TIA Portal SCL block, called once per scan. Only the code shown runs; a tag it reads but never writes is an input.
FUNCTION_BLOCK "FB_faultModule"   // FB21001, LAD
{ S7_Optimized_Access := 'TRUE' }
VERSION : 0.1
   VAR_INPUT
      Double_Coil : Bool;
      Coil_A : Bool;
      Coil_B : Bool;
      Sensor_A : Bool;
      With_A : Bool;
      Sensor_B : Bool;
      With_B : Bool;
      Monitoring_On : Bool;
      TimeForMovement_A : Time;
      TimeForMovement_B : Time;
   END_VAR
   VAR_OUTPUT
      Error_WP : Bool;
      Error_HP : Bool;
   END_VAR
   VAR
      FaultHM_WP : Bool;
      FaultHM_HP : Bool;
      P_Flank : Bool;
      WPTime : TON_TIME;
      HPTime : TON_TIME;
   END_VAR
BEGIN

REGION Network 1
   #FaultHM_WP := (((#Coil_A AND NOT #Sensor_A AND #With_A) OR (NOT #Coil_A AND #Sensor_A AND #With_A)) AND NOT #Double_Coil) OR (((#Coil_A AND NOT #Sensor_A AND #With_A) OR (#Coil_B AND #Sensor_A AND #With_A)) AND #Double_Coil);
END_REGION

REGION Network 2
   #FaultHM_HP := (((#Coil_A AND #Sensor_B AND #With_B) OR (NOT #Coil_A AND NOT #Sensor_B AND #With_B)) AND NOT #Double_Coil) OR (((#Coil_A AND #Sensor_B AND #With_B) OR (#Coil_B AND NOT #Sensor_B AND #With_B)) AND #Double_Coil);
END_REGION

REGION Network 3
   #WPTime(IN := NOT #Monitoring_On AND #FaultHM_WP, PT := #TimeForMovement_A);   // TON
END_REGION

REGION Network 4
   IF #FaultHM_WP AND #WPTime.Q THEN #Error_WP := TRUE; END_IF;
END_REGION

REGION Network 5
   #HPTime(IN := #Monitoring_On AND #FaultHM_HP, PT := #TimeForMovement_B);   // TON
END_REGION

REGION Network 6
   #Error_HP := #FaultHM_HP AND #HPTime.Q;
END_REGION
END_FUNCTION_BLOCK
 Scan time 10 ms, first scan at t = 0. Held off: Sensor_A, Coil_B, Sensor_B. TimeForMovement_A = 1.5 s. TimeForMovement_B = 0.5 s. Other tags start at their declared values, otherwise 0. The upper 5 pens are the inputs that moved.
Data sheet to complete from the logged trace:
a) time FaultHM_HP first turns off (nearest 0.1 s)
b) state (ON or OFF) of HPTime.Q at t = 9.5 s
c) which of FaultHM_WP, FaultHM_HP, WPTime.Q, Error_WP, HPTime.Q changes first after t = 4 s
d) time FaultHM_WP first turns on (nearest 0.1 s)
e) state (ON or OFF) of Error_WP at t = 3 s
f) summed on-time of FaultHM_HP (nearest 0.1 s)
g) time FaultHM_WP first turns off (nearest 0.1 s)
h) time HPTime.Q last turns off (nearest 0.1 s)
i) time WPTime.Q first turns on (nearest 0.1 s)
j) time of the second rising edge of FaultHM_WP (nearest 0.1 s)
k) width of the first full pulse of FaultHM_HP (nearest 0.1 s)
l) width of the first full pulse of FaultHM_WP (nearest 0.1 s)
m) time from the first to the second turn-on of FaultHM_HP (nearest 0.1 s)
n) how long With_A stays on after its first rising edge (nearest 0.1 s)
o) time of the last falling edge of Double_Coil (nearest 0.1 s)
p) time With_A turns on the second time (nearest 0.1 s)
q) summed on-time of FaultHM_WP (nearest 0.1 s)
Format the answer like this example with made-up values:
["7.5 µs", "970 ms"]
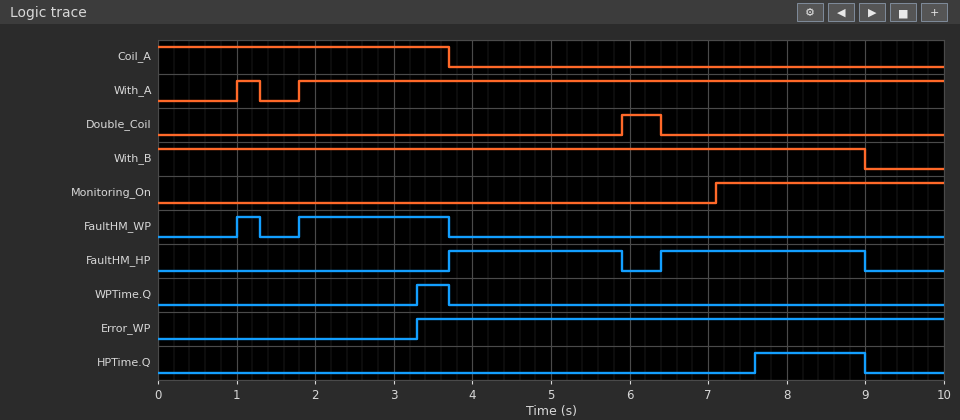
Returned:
["5.9 s", "OFF", "FaultHM_HP", "1.0 s", "OFF", "4.8 s", "1.3 s", "9.0 s", "3.3 s", "1.8 s", "2.2 s", "0.3 s", "2.7 s", "0.3 s", "6.4 s", "1.8 s", "2.2 s"]
